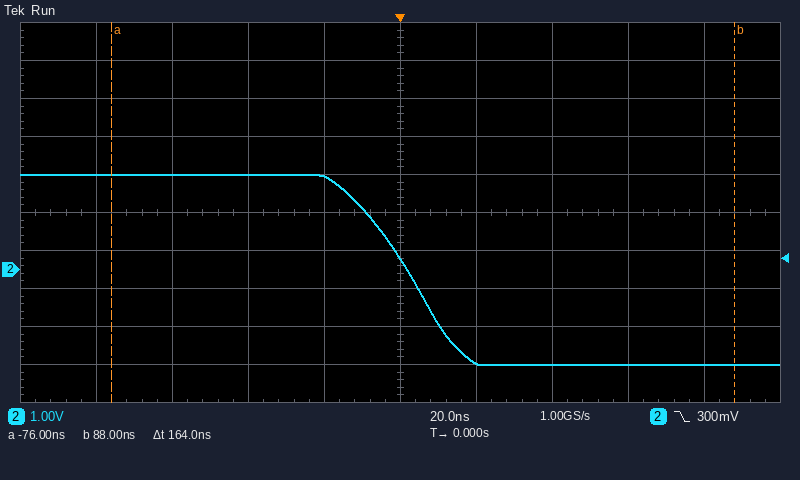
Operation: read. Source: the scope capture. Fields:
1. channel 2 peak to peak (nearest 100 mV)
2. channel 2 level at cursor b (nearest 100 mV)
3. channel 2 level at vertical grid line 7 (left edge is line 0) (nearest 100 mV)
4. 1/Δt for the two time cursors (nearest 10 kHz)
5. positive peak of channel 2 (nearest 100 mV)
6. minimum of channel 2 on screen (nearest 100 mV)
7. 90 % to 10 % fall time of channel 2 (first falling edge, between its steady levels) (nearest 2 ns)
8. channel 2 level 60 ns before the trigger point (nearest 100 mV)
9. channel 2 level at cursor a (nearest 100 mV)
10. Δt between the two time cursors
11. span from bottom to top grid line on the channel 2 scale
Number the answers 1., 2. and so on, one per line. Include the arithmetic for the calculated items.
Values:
1. 2.5 V − (-2.5 V) = 5.0 V
2. -2.5 V
3. -2.5 V
4. 1 / 164 ns ≈ 6.10 MHz
5. 2.5 V
6. -2.5 V
7. 28 ns
8. 2.5 V
9. 2.5 V
10. 164 ns
11. 10 V
